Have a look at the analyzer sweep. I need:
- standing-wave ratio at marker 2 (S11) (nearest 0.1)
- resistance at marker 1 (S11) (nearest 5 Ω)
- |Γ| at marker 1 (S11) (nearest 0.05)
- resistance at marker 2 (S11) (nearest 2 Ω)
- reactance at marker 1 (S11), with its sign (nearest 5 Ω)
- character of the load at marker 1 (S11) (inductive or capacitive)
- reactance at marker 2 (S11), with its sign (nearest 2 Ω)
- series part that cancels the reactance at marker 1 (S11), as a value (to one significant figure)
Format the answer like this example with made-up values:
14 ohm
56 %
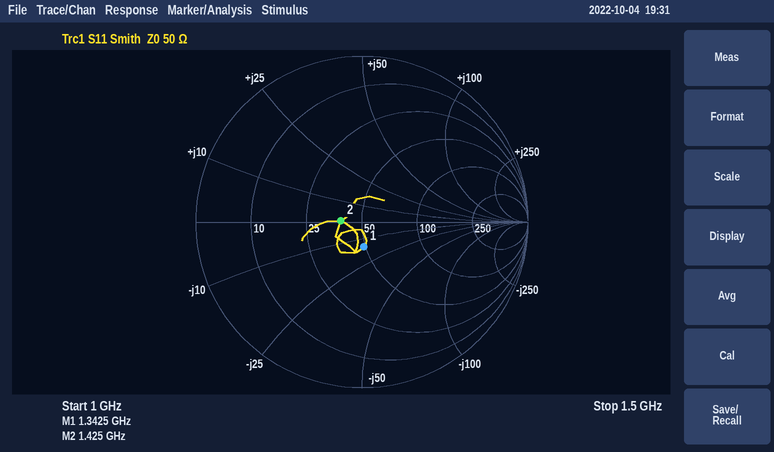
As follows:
1.3
50 Ω
0.15
38 Ω
-15 Ω
capacitive
0 Ω
2 nH
